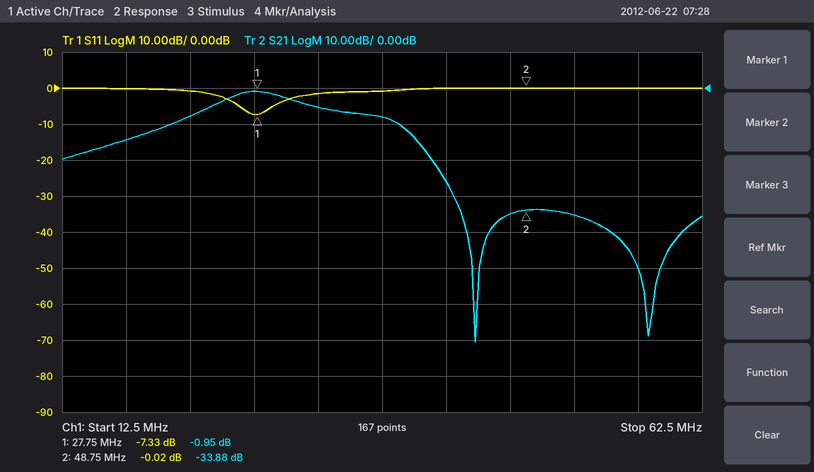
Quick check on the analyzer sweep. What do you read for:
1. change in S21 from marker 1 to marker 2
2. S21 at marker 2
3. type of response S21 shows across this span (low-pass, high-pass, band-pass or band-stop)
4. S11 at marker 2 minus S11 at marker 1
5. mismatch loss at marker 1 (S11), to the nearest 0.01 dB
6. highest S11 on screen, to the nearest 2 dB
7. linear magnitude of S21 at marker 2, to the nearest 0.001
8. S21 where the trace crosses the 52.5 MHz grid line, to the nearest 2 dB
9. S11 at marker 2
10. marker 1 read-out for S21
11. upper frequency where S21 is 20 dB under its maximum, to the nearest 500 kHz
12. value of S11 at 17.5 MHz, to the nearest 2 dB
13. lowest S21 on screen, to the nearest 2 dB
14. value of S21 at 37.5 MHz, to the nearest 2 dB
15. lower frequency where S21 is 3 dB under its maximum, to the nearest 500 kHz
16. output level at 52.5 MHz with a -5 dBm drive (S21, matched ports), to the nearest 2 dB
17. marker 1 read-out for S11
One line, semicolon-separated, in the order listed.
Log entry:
-32.93 dB; -33.88 dB; band-pass; 7.31 dB; 0.89 dB; 0 dB; 0.020; -36 dB; -0.02 dB; -0.95 dB; 41.5 MHz; 0 dB; -70 dB; -8 dB; 25.0 MHz; -40 dBm; -7.33 dB
